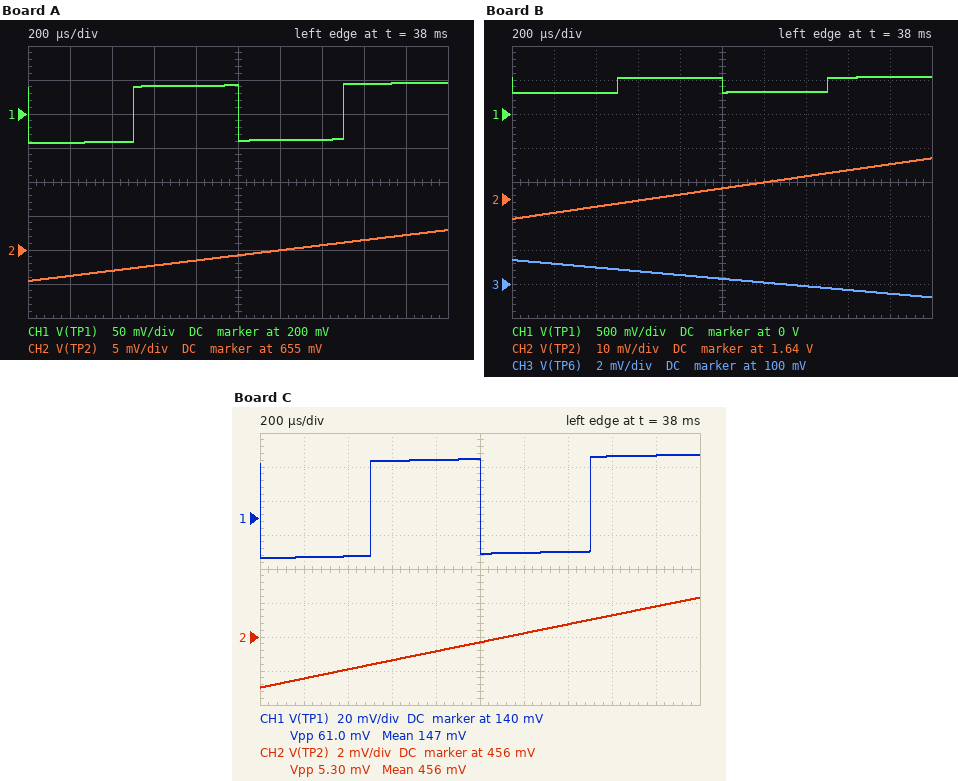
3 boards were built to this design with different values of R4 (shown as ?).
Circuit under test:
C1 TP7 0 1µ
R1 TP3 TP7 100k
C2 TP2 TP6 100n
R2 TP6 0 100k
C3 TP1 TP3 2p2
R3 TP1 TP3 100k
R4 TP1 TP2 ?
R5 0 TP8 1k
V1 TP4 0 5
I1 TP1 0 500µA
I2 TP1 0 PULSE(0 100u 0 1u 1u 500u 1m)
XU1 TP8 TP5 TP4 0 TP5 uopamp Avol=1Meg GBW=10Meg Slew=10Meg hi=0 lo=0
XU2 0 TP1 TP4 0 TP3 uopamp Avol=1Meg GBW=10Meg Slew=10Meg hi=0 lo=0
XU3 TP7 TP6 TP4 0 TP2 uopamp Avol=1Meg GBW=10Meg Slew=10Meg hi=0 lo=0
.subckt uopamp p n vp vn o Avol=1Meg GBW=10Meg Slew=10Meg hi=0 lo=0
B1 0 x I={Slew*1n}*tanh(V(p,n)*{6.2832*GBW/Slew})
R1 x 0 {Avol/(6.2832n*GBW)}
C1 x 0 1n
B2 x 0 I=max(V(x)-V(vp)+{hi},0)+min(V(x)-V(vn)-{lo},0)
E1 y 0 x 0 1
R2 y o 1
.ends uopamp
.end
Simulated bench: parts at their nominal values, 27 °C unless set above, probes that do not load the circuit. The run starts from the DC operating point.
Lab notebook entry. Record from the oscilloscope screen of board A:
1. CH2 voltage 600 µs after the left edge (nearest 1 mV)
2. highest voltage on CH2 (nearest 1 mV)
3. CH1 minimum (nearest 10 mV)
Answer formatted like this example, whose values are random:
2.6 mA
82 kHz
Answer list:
653 mV
658 mV
160 mV
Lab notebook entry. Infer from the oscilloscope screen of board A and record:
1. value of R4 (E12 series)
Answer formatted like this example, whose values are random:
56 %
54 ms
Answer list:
820 Ω
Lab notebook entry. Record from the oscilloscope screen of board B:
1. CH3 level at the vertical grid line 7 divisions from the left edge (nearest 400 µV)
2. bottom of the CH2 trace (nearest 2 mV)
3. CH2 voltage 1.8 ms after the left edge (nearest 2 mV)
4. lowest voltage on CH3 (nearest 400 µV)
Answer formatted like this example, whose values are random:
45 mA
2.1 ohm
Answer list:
100.0 mV
1.634 V
1.650 V
99.2 mV
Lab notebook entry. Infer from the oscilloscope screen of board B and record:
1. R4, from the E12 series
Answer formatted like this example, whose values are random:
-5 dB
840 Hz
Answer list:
2.2 kΩ
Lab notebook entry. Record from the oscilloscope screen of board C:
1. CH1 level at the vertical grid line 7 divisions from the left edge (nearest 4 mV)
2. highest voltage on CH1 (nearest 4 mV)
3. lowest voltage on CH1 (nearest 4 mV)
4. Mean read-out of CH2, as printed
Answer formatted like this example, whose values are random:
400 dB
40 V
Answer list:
120 mV
176 mV
116 mV
456 mV
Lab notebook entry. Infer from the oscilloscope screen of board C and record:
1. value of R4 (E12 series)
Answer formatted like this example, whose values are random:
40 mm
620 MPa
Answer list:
560 Ω
